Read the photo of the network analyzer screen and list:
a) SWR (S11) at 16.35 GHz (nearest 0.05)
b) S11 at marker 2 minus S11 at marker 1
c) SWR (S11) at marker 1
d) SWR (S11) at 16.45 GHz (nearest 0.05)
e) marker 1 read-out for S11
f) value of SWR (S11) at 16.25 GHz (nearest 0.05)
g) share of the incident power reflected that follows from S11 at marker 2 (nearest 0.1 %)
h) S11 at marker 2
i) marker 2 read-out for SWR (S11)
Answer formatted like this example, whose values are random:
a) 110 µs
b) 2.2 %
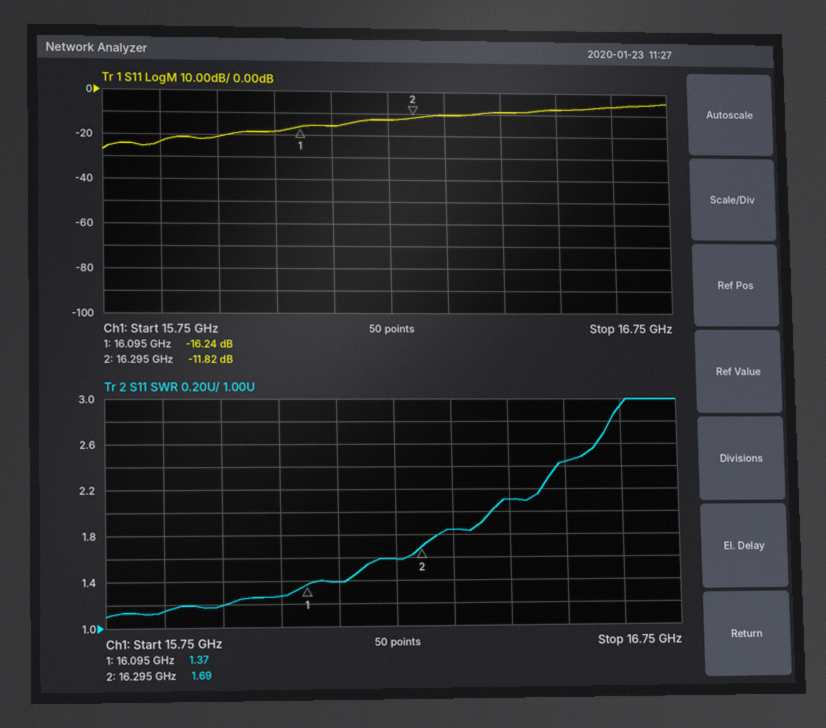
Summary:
a) 1.85
b) 4.42 dB
c) 1.37
d) 2.10
e) -16.24 dB
f) 1.60
g) 6.6 %
h) -11.82 dB
i) 1.69
